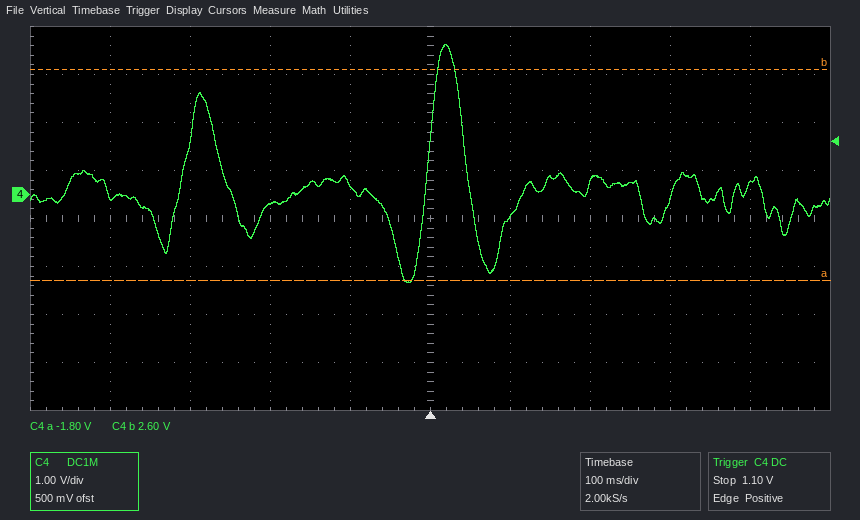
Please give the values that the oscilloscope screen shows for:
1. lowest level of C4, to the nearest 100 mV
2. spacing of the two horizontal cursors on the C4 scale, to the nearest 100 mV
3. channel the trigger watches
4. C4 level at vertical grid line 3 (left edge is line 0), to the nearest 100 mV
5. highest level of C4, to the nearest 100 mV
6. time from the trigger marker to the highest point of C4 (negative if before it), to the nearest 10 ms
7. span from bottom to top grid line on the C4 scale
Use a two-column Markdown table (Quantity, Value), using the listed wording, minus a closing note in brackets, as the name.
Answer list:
| Quantity | Value |
|---|---|
| lowest level of C4, to the nearest 100 mV | -1.8 V |
| spacing of the two horizontal cursors on the C4 scale, to the nearest 100 mV | 4.4 V |
| channel the trigger watches | C4 |
| C4 level at vertical grid line 3 (left edge is line 0), to the nearest 100 mV | -200 mV |
| highest level of C4, to the nearest 100 mV | 3.1 V |
| time from the trigger marker to the highest point of C4 (negative if before it), to the nearest 10 ms | +20 ms |
| span from bottom to top grid line on the C4 scale | 8 V |
